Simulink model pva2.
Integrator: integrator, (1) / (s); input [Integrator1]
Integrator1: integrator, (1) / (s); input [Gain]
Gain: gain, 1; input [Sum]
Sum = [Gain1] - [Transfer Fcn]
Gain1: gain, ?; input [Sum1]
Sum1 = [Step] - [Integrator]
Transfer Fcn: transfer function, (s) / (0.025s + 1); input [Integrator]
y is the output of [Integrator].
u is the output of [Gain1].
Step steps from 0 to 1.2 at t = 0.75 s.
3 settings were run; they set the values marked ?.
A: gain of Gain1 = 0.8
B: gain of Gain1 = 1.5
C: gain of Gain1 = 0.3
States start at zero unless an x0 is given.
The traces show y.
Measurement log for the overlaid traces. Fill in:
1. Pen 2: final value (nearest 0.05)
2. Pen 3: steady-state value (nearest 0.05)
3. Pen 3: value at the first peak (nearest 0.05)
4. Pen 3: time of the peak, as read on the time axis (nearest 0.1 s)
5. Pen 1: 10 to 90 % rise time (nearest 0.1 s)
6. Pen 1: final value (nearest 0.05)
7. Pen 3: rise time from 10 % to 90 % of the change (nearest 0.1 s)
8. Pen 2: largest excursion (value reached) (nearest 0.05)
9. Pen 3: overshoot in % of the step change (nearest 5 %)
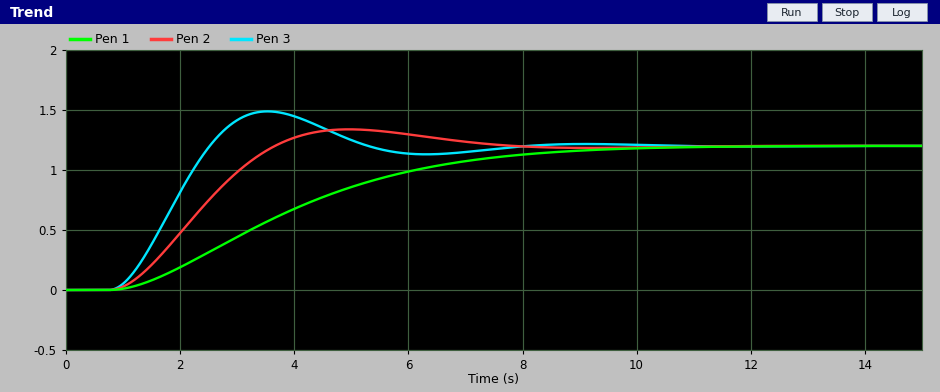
1.20
1.20
1.50
3.5 s
5.4 s
1.20
1.2 s
1.35
25 %
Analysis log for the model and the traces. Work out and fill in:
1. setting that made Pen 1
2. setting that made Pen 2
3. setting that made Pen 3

C
A
B
